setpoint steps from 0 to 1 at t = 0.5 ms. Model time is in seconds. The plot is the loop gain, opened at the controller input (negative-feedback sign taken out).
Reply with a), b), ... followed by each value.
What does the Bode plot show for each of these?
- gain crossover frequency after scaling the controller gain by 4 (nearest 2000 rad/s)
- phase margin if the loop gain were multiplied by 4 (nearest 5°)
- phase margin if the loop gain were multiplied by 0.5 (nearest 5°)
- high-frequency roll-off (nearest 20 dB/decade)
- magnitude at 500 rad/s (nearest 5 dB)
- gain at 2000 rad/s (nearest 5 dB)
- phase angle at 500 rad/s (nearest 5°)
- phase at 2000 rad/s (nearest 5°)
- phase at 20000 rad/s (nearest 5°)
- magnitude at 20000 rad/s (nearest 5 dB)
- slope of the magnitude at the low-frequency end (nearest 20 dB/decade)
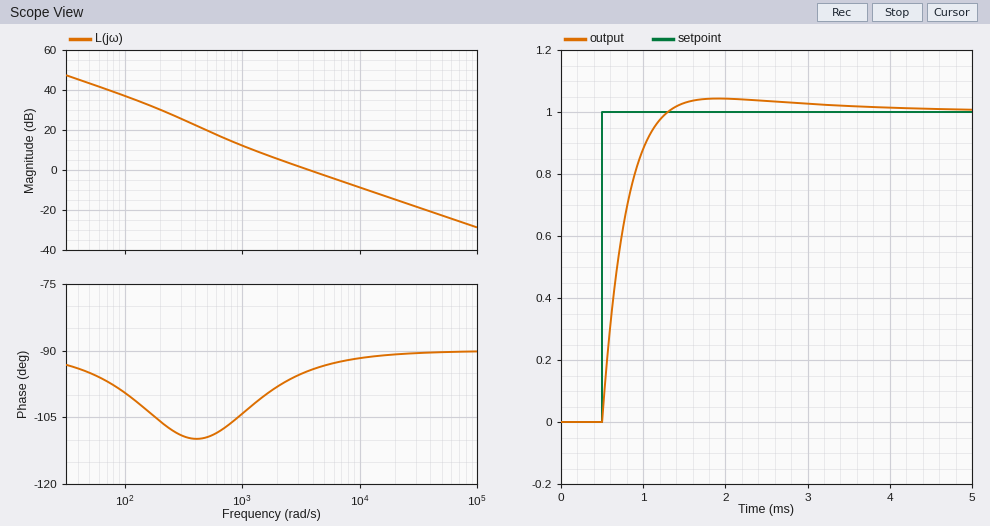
a) 14000 rad/s
b) 90°
c) 80°
d) -20 dB/decade
e) 20 dB
f) 5 dB
g) -110°
h) -100°
i) -90°
j) -15 dB
k) -20 dB/decade
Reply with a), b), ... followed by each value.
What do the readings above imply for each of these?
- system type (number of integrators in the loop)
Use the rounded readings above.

a) 1
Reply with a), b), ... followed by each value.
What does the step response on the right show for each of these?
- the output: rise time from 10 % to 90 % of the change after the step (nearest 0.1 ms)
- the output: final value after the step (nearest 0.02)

a) 0.5 ms
b) 1.00
